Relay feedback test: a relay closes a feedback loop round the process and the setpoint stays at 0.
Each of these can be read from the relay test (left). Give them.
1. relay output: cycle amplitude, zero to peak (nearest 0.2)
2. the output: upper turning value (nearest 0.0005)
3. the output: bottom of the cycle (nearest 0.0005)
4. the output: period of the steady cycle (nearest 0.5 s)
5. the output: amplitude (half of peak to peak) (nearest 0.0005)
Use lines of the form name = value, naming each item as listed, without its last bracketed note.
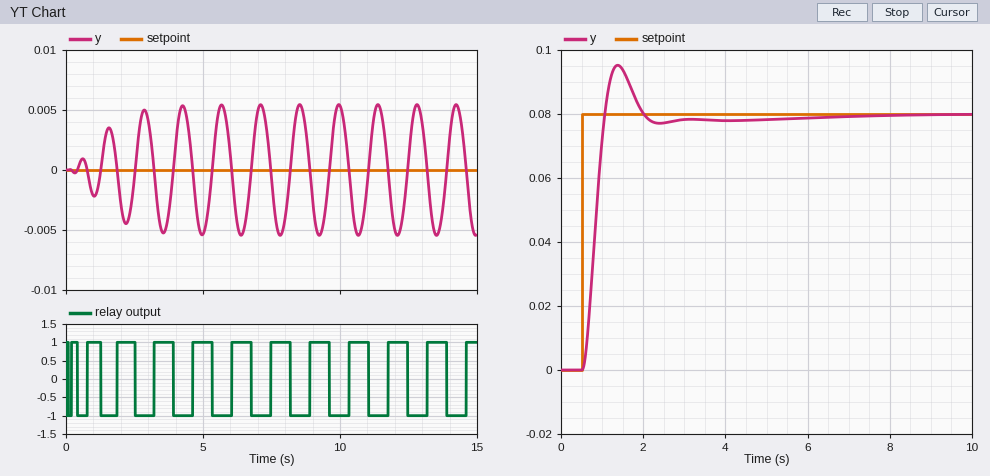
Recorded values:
relay output: cycle amplitude, zero to peak = 1.0
the output: upper turning value = 0.0055
the output: bottom of the cycle = -0.0055
the output: period of the steady cycle = 1.5 s
the output: amplitude (half of peak to peak) = 0.0055
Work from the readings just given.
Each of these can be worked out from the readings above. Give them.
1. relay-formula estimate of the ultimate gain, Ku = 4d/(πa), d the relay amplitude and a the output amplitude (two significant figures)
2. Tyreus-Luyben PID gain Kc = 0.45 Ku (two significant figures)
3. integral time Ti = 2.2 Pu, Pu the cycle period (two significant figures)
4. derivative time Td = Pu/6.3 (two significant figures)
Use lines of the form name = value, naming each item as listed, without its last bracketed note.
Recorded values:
relay-formula estimate of the ultimate gain, Ku = 4d/(πa), d the relay amplitude and a the output amplitude = 230
Tyreus-Luyben PID gain Kc = 0.45 Ku = 100
integral time Ti = 2.2 Pu, Pu the cycle period = 3.3 s
derivative time Td = Pu/6.3 = 0.24 s
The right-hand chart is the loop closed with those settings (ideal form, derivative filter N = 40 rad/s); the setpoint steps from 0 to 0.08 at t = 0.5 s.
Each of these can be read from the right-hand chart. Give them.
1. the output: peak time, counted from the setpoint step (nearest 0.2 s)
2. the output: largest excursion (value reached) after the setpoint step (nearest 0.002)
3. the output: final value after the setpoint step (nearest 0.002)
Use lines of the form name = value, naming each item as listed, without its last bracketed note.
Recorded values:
the output: peak time, counted from the setpoint step = 0.8 s
the output: largest excursion (value reached) after the setpoint step = 0.096
the output: final value after the setpoint step = 0.080
